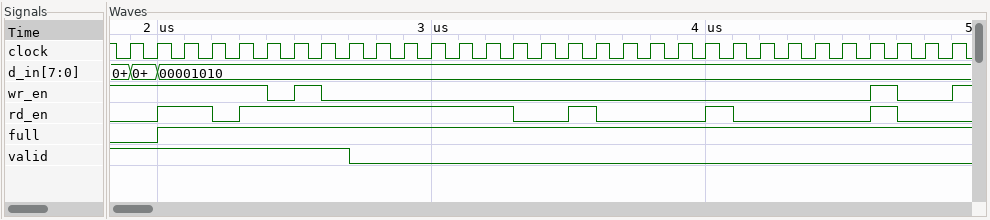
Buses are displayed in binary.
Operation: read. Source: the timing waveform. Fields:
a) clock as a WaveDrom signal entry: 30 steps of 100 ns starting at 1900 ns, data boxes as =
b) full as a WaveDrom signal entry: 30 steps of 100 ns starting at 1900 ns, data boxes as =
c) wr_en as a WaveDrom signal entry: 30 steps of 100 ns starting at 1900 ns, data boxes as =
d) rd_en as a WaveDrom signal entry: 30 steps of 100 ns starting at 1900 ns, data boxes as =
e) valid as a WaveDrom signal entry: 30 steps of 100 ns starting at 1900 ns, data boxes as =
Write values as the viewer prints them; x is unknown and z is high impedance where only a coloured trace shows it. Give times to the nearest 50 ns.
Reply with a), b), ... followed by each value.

a) {name: 'clock', wave: 'p.............................'}
b) {name: 'full', wave: '01............................'}
c) {name: 'wr_en', wave: '1....010...................10.'}
d) {name: 'rd_en', wave: '01.01.........0.10...10....10.'}
e) {name: 'valid', wave: '1.......0.....................'}
